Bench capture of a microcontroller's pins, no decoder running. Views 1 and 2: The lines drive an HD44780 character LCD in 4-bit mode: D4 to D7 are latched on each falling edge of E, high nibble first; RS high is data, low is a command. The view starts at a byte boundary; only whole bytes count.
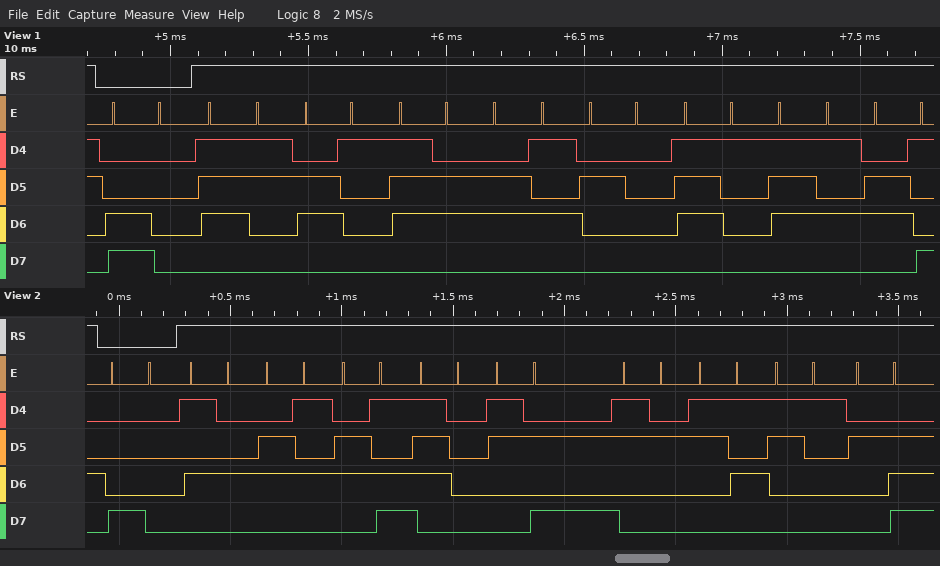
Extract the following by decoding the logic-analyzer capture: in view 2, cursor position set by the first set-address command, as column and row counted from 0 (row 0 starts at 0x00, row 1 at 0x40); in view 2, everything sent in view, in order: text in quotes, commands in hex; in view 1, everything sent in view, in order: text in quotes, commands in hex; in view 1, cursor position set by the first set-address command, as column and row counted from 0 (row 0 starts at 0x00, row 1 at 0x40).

column 0, row 0
0x80 "Temp:251."
0xC0 "save qui"
column 0, row 1
